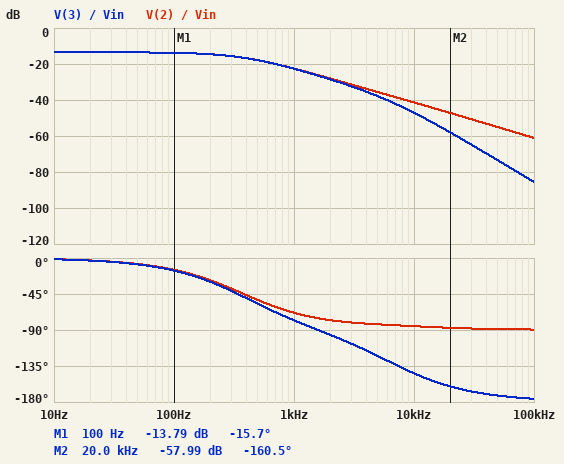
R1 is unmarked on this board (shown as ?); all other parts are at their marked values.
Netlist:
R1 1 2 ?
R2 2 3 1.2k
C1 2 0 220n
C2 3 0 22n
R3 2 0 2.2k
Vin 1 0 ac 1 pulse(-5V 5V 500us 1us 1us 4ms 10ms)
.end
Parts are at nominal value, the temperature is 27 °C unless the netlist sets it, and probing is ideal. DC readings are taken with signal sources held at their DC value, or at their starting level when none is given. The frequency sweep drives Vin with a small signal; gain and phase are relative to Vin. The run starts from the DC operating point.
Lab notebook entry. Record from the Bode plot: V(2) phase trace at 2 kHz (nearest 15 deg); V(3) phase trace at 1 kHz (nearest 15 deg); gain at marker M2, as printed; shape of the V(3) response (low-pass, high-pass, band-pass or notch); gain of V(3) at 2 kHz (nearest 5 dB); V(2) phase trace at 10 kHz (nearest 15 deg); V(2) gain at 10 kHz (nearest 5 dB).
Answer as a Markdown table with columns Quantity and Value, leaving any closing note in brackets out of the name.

| Quantity | Value |
|---|---|
| V(2) phase trace at 2 kHz | -75 deg |
| V(3) phase trace at 1 kHz | -75 deg |
| gain at marker M2, as printed | -57.99 dB |
| shape of the V(3) response | low-pass |
| gain of V(3) at 2 kHz | -30 dB |
| V(2) phase trace at 10 kHz | -90 deg |
| V(2) gain at 10 kHz | -40 dB |
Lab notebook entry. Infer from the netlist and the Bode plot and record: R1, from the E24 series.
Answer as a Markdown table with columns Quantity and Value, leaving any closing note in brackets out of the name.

| Quantity | Value |
|---|---|
| R1, from the E24 series | 8.2 kΩ |
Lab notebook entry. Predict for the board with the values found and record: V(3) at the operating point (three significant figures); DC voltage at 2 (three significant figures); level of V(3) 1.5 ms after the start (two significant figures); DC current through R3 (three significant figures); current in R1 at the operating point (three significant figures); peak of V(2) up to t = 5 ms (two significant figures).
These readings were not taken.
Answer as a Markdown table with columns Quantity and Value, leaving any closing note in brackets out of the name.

| Quantity | Value |
|---|---|
| V(3) at the operating point | -1.06 V |
| DC voltage at 2 | -1.06 V |
| level of V(3) 1.5 ms after the start | 850 mV |
| DC current through R3 | 481 µA |
| current in R1 at the operating point | 481 µA |
| peak of V(2) up to t = 5 ms | 1.1 V |
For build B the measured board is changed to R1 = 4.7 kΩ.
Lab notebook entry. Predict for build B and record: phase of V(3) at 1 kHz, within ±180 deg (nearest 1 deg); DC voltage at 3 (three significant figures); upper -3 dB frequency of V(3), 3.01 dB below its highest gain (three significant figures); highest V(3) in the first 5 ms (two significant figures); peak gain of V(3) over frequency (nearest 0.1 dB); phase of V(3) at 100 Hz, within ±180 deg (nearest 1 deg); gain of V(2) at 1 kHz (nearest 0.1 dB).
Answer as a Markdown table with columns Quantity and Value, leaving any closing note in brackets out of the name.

| Quantity | Value |
|---|---|
| phase of V(3) at 1 kHz, within ±180 deg | -75 deg |
| DC voltage at 3 | -1.59 V |
| upper -3 dB frequency of V(3), 3.01 dB below its highest gain | 434 Hz |
| highest V(3) in the first 5 ms | 1.6 V |
| peak gain of V(3) over frequency | -9.9 dB |
| phase of V(3) at 100 Hz, within ±180 deg | -14 deg |
| gain of V(2) at 1 kHz | -17.9 dB |
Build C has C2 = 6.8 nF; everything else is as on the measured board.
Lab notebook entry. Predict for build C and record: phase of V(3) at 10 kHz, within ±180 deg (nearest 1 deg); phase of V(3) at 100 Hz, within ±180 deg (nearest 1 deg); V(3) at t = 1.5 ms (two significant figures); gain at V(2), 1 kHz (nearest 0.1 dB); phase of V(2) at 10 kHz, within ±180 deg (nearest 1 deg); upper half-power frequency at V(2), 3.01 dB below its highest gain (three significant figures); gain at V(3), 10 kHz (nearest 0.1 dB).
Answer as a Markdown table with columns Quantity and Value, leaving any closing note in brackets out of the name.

| Quantity | Value |
|---|---|
| phase of V(3) at 10 kHz, within ±180 deg | -114 deg |
| phase of V(3) at 100 Hz, within ±180 deg | -14 deg |
| V(3) at t = 1.5 ms | 890 mV |
| gain at V(2), 1 kHz | -22.0 dB |
| phase of V(2) at 10 kHz, within ±180 deg | -87 deg |
| upper half-power frequency at V(2), 3.01 dB below its highest gain | 404 Hz |
| gain at V(3), 10 kHz | -42.3 dB |
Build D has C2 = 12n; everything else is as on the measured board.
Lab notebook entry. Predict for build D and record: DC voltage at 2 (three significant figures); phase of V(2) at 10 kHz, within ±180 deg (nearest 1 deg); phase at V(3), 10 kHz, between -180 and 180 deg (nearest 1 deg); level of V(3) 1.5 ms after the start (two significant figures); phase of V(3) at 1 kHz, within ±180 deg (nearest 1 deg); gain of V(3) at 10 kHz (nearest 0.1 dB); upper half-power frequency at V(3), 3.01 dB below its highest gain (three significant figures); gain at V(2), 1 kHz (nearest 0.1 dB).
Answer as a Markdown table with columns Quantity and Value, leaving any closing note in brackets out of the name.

| Quantity | Value |
|---|---|
| DC voltage at 2 | -1.06 V |
| phase of V(2) at 10 kHz, within ±180 deg | -86 deg |
| phase at V(3), 10 kHz, between -180 and 180 deg | -128 deg |
| level of V(3) 1.5 ms after the start | 870 mV |
| phase of V(3) at 1 kHz, within ±180 deg | -73 deg |
| gain of V(3) at 10 kHz | -44.0 dB |
| upper half-power frequency at V(3), 3.01 dB below its highest gain | 394 Hz |
| gain at V(2), 1 kHz | -22.2 dB |
